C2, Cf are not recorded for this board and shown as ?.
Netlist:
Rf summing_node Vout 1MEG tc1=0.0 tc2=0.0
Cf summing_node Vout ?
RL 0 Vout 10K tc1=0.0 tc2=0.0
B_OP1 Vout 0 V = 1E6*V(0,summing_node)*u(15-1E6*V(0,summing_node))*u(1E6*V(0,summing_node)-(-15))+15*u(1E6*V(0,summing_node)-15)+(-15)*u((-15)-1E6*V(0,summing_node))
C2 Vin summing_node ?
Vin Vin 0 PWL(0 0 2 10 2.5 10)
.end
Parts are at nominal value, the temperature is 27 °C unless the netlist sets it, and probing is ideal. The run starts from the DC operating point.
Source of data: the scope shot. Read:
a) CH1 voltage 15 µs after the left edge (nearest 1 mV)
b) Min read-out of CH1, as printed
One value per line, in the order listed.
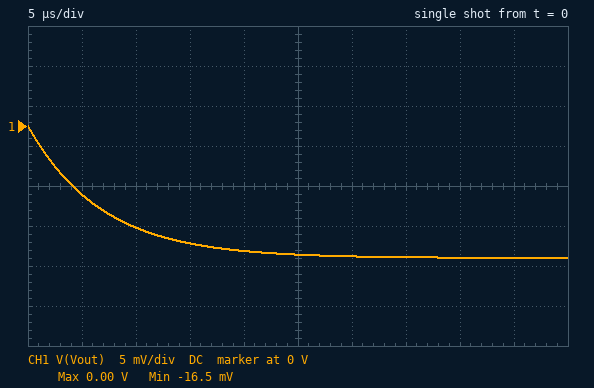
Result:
-15 mV
-16.5 mV
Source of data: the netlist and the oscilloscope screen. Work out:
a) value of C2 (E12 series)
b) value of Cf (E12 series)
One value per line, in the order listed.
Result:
3.3 nF
6.8 pF
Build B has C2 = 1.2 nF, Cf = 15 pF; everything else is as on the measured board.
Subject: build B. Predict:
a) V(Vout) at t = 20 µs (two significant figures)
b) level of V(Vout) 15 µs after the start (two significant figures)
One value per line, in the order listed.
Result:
-4.4 mV
-3.8 mV
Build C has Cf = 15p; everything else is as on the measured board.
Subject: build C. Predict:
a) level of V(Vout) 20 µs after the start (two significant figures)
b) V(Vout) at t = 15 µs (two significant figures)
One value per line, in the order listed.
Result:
-12 mV
-10 mV
